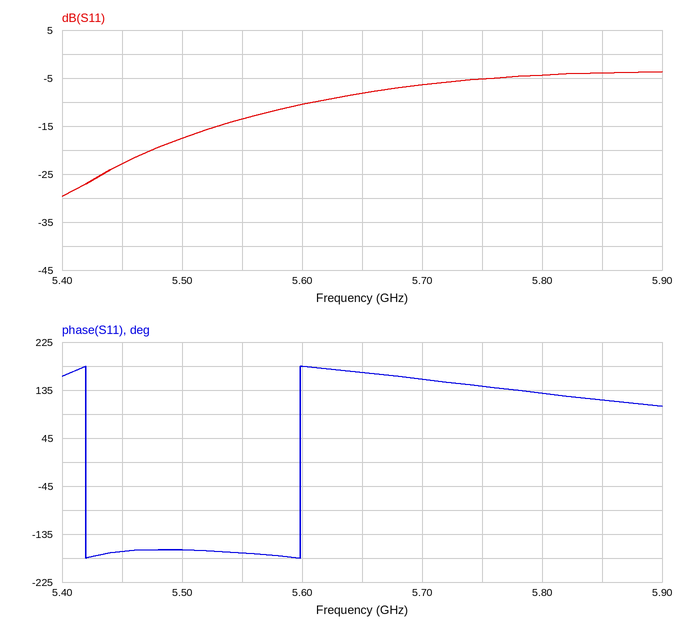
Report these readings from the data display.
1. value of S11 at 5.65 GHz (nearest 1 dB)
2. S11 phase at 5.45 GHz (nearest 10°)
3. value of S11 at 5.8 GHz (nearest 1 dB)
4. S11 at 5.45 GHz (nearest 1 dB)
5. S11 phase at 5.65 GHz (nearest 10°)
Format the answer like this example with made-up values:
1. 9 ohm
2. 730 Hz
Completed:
1. -8 dB
2. -170°
3. -4 dB
4. -23 dB
5. 170°
